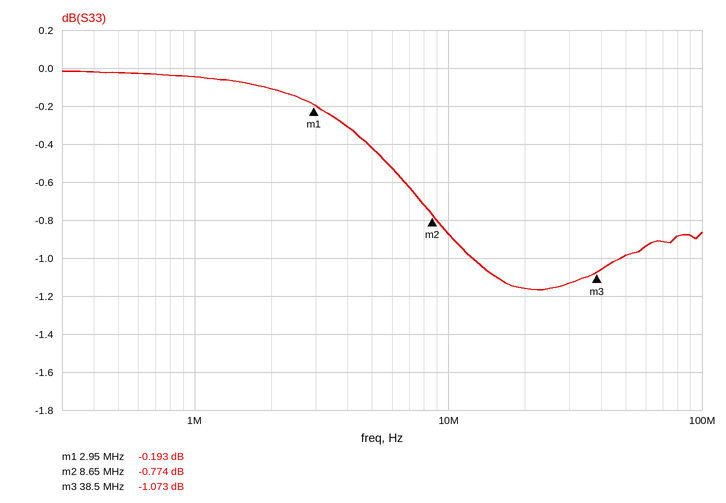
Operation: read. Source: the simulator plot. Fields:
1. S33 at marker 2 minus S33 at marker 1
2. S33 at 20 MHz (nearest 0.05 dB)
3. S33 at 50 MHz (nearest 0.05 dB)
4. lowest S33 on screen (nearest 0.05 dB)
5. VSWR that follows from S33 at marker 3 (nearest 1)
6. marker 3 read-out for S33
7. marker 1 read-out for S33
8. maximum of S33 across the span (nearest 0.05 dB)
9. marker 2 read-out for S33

-0.581 dB
-1.15 dB
-1.00 dB
-1.15 dB
16
-1.073 dB
-0.193 dB
0.00 dB
-0.774 dB
